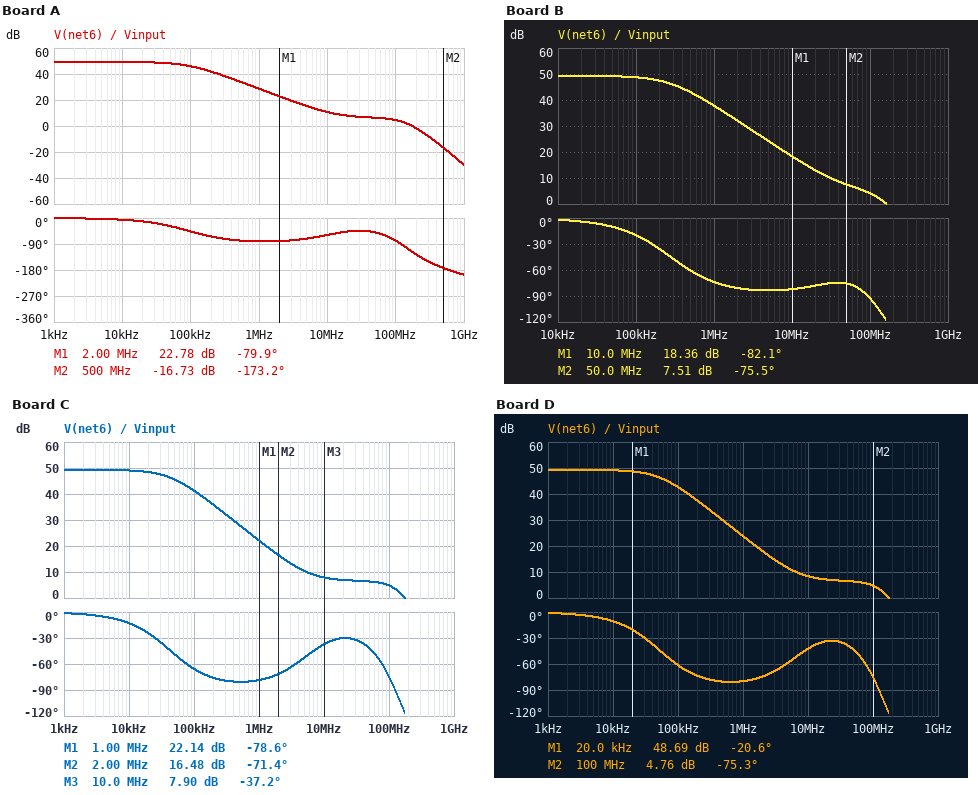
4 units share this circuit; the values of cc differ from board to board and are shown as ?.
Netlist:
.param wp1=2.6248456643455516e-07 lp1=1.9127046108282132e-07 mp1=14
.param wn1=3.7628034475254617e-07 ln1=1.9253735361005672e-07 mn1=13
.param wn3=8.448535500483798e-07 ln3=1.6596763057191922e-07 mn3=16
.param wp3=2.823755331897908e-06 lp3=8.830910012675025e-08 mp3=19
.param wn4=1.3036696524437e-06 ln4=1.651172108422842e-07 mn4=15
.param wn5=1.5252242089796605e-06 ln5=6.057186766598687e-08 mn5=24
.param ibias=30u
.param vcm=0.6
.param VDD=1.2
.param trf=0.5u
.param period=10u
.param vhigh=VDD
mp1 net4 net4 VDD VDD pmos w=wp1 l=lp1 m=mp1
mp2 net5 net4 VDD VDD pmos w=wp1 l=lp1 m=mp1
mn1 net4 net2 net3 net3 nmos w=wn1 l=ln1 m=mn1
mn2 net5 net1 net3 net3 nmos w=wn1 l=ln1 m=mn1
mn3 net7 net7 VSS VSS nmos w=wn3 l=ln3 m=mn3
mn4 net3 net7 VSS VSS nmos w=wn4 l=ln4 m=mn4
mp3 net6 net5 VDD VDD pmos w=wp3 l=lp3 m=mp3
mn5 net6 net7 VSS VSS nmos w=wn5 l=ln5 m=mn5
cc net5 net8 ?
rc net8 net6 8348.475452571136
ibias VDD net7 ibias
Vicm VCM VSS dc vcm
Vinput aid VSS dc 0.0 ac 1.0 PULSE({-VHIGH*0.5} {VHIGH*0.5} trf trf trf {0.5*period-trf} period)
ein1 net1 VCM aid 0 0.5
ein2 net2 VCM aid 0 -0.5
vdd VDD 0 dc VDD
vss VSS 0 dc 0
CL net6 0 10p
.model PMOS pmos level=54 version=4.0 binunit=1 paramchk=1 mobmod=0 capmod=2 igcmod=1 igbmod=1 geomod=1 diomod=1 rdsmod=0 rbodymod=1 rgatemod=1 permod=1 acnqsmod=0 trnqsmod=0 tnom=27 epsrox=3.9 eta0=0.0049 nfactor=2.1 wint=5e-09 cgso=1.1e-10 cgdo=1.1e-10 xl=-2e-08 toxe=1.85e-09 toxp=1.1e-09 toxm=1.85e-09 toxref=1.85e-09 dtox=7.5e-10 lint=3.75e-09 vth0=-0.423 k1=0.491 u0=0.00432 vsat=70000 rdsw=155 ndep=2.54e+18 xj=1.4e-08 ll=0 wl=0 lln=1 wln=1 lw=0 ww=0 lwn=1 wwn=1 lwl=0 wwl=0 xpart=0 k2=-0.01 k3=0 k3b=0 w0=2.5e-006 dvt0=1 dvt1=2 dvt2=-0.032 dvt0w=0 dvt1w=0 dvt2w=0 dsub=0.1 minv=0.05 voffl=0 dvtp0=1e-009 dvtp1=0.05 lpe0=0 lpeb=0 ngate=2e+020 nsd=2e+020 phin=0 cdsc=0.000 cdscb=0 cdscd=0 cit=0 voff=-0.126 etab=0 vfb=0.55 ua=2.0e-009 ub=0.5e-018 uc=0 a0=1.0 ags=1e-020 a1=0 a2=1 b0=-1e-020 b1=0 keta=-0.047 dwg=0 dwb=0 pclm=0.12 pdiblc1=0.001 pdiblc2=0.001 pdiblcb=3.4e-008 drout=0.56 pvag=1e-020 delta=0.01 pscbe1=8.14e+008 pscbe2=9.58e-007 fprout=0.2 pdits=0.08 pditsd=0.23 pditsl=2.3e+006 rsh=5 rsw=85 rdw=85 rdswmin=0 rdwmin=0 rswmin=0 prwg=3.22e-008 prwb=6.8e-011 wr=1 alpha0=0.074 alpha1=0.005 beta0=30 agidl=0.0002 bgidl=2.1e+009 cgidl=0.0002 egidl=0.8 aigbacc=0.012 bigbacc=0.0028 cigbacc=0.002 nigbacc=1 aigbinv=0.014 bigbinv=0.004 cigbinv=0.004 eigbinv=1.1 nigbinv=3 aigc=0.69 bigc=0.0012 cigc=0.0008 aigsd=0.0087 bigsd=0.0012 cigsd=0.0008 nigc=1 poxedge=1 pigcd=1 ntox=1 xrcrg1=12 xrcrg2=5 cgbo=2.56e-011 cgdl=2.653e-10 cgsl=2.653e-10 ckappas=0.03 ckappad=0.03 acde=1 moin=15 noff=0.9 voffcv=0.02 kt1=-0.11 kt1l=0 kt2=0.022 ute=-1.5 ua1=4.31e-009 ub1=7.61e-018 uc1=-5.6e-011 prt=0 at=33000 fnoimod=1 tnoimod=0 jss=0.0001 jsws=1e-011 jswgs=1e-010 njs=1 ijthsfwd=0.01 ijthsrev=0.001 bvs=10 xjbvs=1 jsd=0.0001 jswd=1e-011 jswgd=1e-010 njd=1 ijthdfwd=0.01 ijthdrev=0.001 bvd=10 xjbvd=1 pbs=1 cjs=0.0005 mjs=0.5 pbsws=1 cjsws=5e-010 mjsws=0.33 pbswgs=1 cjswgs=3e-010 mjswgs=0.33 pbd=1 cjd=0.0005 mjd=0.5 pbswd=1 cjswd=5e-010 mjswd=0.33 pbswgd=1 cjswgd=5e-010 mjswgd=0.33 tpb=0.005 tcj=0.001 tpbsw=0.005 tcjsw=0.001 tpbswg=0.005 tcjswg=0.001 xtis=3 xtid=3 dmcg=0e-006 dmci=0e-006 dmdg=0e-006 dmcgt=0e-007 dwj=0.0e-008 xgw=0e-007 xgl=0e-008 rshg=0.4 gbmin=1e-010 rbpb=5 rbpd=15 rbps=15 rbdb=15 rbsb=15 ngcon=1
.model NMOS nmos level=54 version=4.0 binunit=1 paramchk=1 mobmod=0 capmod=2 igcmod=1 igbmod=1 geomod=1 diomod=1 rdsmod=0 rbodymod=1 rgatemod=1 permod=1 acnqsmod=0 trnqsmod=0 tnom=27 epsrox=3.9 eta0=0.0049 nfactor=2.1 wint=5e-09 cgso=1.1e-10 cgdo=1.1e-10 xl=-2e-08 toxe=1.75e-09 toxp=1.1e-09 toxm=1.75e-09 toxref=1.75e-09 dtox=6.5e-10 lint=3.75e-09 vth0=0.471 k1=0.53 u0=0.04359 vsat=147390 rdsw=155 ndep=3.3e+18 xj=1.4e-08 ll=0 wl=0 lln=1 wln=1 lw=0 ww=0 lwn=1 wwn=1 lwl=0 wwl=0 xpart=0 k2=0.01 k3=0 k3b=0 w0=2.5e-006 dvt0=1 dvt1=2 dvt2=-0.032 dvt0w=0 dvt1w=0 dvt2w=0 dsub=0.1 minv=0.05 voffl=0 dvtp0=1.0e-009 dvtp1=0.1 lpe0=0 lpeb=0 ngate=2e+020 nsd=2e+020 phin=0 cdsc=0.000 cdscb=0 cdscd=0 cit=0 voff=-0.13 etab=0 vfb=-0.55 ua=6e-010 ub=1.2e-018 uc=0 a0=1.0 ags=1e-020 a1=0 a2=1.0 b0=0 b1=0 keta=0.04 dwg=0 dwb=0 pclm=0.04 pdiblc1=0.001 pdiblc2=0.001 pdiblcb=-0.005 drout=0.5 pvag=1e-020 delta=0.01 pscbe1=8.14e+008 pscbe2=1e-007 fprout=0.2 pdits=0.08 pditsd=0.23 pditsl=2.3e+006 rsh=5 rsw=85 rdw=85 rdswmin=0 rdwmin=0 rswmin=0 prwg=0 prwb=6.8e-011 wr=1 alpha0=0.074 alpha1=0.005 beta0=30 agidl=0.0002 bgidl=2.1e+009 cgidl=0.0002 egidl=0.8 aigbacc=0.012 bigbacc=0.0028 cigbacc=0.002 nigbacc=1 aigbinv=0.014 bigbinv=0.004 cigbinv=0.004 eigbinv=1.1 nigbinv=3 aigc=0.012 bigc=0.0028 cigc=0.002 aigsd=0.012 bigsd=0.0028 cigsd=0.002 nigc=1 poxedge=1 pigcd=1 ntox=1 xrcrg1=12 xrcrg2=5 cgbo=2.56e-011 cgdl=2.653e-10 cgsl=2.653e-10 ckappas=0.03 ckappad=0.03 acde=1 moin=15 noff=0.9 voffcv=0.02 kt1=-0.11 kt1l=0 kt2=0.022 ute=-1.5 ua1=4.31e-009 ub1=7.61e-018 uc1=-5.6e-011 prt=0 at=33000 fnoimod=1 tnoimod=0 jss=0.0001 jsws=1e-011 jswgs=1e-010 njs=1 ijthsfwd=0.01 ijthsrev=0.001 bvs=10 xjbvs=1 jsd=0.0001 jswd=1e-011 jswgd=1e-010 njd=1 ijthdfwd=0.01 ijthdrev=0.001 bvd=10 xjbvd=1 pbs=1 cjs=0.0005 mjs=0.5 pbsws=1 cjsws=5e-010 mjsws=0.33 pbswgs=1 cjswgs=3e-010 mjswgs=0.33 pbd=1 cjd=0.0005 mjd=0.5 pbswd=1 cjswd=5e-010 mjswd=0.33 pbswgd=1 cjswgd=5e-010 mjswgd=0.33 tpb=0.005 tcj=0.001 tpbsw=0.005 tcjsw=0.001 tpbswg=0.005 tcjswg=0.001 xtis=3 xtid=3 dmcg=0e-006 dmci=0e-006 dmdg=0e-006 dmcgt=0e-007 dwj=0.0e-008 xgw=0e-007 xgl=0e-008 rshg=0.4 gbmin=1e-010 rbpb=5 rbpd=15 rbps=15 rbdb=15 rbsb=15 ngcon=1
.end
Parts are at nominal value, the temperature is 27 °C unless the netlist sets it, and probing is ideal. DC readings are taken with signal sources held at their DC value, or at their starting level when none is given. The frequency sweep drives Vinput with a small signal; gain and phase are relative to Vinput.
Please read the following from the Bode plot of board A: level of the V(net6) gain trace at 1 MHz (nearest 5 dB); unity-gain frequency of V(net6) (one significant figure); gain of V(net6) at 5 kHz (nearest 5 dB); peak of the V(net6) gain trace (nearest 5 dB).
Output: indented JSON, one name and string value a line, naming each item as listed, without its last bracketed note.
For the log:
{
  "level of the V(net6) gain trace at 1 MHz": "30 dB",
  "unity-gain frequency of V(net6)": "200 MHz",
  "gain of V(net6) at 5 kHz": "50 dB",
  "peak of the V(net6) gain trace": "50 dB"
}
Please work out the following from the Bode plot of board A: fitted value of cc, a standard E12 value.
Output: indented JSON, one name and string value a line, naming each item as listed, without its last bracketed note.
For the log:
{
  "fitted value of cc, a standard E12 value": "1.5 pF"
}
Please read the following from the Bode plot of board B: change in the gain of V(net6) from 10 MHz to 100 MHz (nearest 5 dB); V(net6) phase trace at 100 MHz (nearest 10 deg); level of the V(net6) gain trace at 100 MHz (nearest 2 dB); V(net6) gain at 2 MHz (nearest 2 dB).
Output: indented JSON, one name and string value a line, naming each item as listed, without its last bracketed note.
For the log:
{
  "change in the gain of V(net6) from 10 MHz to 100 MHz": "-15 dB",
  "V(net6) phase trace at 100 MHz": "-90 deg",
  "level of the V(net6) gain trace at 100 MHz": "4 dB",
  "V(net6) gain at 2 MHz": "32 dB"
}
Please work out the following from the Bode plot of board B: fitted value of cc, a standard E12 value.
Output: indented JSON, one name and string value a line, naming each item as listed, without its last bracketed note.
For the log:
{
  "fitted value of cc, a standard E12 value": "470 fF"
}
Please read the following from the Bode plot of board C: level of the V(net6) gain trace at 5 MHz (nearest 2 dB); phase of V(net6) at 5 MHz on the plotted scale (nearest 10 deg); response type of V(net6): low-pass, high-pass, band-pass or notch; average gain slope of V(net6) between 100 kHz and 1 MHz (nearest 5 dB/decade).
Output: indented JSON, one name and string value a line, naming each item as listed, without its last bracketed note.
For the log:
{
  "level of the V(net6) gain trace at 5 MHz": "10 dB",
  "phase of V(net6) at 5 MHz on the plotted scale": "-50 deg",
  "response type of V(net6): low-pass, high-pass, band-pass or notch": "low-pass",
  "average gain slope of V(net6) between 100 kHz and 1 MHz": "-20 dB/decade"
}
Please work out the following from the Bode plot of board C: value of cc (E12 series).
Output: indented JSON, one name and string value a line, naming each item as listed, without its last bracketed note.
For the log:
{
  "value of cc": "3.3 pF"
}
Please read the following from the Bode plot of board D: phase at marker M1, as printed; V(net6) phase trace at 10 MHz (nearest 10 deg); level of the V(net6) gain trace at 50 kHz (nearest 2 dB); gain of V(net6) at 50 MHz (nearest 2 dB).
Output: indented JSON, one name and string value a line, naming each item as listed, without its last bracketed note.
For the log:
{
  "phase at marker M1, as printed": "-20.6 deg",
  "V(net6) phase trace at 10 MHz": "-40 deg",
  "level of the V(net6) gain trace at 50 kHz": "46 dB",
  "gain of V(net6) at 50 MHz": "6 dB"
}
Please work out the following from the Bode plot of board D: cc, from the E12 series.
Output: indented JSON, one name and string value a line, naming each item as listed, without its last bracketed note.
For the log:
{
  "cc, from the E12 series": "2.7 pF"
}
